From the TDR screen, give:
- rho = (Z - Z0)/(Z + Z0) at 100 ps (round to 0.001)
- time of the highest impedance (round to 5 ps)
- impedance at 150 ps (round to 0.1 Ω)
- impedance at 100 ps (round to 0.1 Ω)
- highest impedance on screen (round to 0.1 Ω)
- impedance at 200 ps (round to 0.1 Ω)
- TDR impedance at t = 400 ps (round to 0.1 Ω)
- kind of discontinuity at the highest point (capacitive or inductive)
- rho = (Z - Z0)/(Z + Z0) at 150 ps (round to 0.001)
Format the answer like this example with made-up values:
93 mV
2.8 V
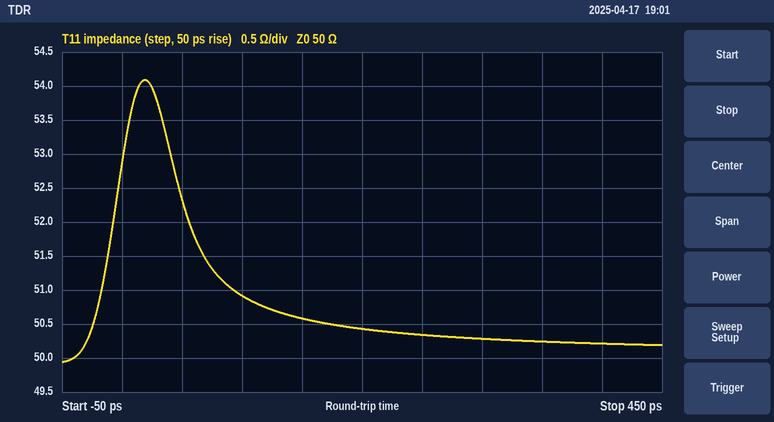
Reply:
+0.009
20 ps
50.6 Ω
50.9 Ω
54.1 Ω
50.4 Ω
50.2 Ω
inductive
+0.006
